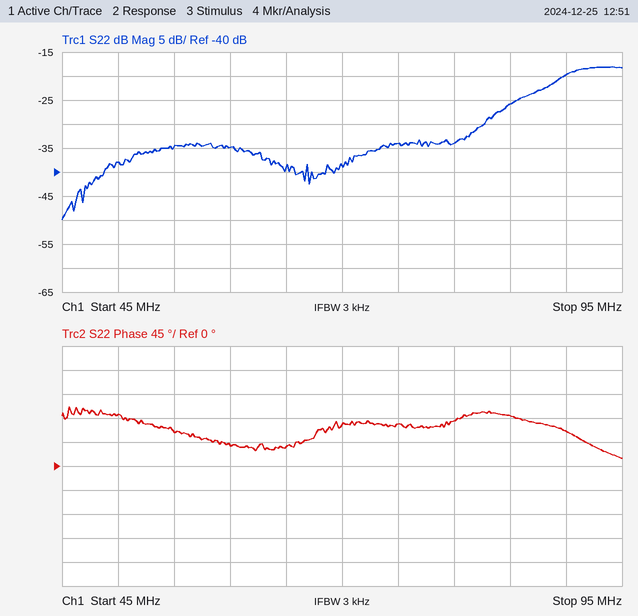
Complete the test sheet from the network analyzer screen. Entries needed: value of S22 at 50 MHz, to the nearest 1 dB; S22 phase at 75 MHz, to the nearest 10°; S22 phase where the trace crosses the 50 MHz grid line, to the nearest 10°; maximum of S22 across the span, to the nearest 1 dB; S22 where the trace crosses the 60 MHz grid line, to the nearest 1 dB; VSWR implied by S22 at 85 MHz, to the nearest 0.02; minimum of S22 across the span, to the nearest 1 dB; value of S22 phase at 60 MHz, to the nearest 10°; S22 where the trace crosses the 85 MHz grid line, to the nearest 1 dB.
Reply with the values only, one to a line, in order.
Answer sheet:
-38 dB
80°
100°
-18 dB
-35 dB
1.10
-50 dB
40°
-26 dB
